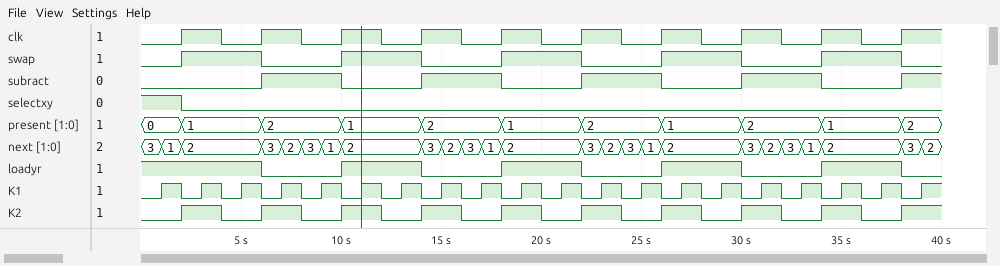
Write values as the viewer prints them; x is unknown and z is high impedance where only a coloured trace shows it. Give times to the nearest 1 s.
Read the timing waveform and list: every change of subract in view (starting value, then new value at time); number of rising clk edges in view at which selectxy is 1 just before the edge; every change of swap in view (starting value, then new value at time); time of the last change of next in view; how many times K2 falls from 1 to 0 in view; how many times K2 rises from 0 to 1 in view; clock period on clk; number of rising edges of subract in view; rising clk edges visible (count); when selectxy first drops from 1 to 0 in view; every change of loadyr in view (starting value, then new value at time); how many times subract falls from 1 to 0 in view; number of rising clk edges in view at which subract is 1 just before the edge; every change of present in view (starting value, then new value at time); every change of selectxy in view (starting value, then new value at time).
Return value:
0, 1 at 6 s, 0 at 10 s, 1 at 14 s, 0 at 18 s, 1 at 22 s, 0 at 26 s, 1 at 30 s, 0 at 34 s, 1 at 38 s
1
0, 1 at 2 s, 0 at 6 s, 1 at 10 s, 0 at 14 s, 1 at 18 s, 0 at 22 s, 1 at 26 s, 0 at 30 s, 1 at 34 s, 0 at 38 s
39 s
9
10
4 s
5
10
2 s
1, 0 at 6 s, 1 at 10 s, 0 at 14 s, 1 at 18 s, 0 at 22 s, 1 at 26 s, 0 at 30 s, 1 at 34 s, 0 at 38 s
4
4
0, 1 at 2 s, 2 at 6 s, 1 at 10 s, 2 at 14 s, 1 at 18 s, 2 at 22 s, 1 at 26 s, 2 at 30 s, 1 at 34 s, 2 at 38 s
1, 0 at 2 s
